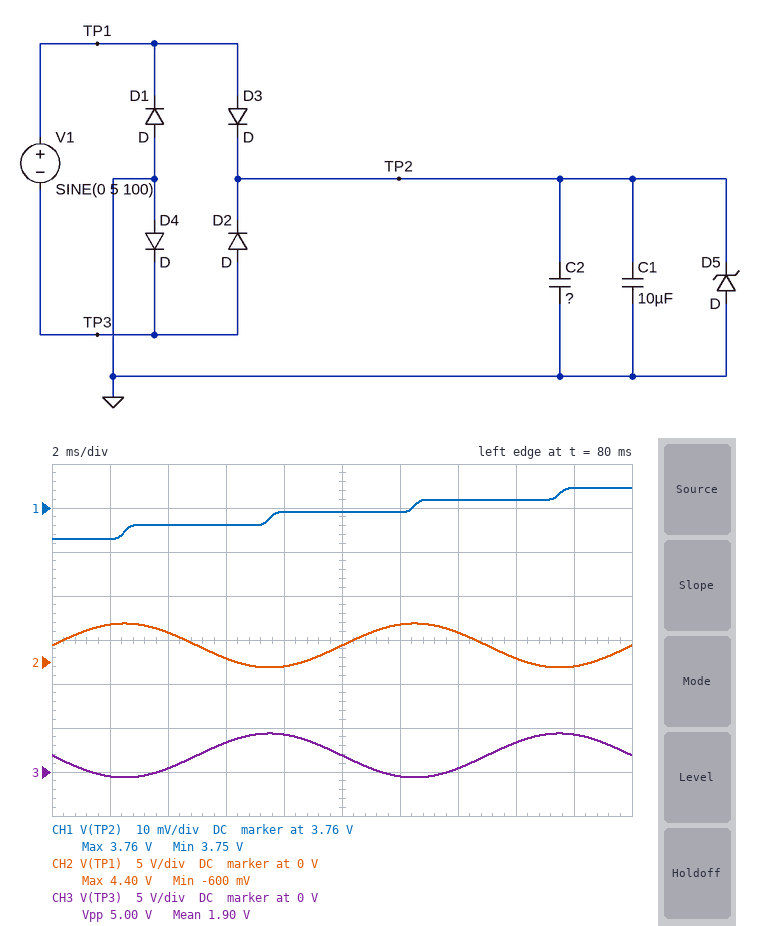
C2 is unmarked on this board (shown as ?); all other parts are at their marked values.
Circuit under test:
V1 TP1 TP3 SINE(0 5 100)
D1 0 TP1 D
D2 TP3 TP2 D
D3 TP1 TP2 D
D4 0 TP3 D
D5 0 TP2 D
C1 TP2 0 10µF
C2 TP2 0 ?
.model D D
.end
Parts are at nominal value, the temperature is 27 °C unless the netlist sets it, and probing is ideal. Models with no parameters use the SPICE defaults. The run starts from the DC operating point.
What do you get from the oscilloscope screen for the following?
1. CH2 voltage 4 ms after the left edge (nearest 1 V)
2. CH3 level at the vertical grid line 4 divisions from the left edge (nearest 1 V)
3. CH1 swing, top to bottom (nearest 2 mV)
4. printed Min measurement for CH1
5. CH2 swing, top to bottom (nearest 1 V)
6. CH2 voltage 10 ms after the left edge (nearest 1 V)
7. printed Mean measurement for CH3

3 V
4 V
12 mV
3.75 V
5 V
2 V
1.90 V
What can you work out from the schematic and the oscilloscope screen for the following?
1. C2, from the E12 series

27 µF
